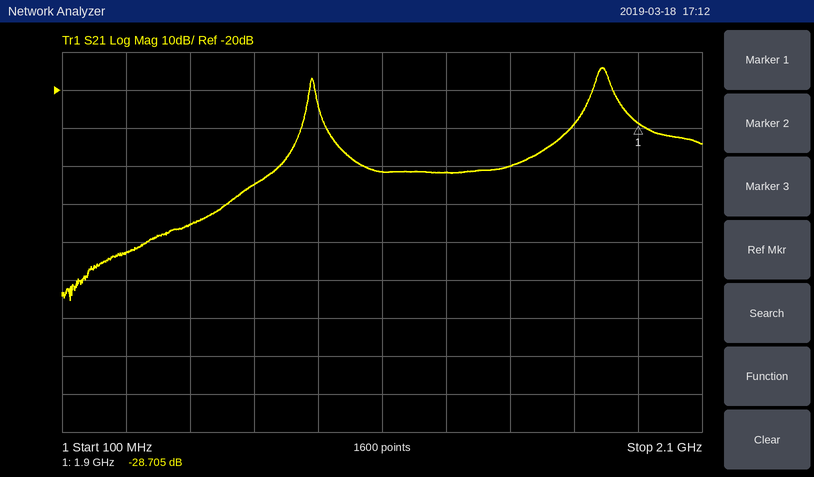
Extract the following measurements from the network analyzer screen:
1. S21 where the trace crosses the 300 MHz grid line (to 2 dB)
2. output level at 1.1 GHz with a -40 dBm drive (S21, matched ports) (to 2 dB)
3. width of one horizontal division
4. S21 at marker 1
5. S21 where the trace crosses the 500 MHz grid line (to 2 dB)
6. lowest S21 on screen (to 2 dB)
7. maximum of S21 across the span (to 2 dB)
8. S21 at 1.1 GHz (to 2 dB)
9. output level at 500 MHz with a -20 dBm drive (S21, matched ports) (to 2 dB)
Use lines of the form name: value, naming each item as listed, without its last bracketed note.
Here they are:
S21 where the trace crosses the 300 MHz grid line: -62 dB
output level at 1.1 GHz with a -40 dBm drive (S21, matched ports): -82 dBm
width of one horizontal division: 200 MHz
S21 at marker 1: -28.705 dB
S21 where the trace crosses the 500 MHz grid line: -56 dB
lowest S21 on screen: -76 dB
maximum of S21 across the span: -14 dB
S21 at 1.1 GHz: -42 dB
output level at 500 MHz with a -20 dBm drive (S21, matched ports): -76 dBm
